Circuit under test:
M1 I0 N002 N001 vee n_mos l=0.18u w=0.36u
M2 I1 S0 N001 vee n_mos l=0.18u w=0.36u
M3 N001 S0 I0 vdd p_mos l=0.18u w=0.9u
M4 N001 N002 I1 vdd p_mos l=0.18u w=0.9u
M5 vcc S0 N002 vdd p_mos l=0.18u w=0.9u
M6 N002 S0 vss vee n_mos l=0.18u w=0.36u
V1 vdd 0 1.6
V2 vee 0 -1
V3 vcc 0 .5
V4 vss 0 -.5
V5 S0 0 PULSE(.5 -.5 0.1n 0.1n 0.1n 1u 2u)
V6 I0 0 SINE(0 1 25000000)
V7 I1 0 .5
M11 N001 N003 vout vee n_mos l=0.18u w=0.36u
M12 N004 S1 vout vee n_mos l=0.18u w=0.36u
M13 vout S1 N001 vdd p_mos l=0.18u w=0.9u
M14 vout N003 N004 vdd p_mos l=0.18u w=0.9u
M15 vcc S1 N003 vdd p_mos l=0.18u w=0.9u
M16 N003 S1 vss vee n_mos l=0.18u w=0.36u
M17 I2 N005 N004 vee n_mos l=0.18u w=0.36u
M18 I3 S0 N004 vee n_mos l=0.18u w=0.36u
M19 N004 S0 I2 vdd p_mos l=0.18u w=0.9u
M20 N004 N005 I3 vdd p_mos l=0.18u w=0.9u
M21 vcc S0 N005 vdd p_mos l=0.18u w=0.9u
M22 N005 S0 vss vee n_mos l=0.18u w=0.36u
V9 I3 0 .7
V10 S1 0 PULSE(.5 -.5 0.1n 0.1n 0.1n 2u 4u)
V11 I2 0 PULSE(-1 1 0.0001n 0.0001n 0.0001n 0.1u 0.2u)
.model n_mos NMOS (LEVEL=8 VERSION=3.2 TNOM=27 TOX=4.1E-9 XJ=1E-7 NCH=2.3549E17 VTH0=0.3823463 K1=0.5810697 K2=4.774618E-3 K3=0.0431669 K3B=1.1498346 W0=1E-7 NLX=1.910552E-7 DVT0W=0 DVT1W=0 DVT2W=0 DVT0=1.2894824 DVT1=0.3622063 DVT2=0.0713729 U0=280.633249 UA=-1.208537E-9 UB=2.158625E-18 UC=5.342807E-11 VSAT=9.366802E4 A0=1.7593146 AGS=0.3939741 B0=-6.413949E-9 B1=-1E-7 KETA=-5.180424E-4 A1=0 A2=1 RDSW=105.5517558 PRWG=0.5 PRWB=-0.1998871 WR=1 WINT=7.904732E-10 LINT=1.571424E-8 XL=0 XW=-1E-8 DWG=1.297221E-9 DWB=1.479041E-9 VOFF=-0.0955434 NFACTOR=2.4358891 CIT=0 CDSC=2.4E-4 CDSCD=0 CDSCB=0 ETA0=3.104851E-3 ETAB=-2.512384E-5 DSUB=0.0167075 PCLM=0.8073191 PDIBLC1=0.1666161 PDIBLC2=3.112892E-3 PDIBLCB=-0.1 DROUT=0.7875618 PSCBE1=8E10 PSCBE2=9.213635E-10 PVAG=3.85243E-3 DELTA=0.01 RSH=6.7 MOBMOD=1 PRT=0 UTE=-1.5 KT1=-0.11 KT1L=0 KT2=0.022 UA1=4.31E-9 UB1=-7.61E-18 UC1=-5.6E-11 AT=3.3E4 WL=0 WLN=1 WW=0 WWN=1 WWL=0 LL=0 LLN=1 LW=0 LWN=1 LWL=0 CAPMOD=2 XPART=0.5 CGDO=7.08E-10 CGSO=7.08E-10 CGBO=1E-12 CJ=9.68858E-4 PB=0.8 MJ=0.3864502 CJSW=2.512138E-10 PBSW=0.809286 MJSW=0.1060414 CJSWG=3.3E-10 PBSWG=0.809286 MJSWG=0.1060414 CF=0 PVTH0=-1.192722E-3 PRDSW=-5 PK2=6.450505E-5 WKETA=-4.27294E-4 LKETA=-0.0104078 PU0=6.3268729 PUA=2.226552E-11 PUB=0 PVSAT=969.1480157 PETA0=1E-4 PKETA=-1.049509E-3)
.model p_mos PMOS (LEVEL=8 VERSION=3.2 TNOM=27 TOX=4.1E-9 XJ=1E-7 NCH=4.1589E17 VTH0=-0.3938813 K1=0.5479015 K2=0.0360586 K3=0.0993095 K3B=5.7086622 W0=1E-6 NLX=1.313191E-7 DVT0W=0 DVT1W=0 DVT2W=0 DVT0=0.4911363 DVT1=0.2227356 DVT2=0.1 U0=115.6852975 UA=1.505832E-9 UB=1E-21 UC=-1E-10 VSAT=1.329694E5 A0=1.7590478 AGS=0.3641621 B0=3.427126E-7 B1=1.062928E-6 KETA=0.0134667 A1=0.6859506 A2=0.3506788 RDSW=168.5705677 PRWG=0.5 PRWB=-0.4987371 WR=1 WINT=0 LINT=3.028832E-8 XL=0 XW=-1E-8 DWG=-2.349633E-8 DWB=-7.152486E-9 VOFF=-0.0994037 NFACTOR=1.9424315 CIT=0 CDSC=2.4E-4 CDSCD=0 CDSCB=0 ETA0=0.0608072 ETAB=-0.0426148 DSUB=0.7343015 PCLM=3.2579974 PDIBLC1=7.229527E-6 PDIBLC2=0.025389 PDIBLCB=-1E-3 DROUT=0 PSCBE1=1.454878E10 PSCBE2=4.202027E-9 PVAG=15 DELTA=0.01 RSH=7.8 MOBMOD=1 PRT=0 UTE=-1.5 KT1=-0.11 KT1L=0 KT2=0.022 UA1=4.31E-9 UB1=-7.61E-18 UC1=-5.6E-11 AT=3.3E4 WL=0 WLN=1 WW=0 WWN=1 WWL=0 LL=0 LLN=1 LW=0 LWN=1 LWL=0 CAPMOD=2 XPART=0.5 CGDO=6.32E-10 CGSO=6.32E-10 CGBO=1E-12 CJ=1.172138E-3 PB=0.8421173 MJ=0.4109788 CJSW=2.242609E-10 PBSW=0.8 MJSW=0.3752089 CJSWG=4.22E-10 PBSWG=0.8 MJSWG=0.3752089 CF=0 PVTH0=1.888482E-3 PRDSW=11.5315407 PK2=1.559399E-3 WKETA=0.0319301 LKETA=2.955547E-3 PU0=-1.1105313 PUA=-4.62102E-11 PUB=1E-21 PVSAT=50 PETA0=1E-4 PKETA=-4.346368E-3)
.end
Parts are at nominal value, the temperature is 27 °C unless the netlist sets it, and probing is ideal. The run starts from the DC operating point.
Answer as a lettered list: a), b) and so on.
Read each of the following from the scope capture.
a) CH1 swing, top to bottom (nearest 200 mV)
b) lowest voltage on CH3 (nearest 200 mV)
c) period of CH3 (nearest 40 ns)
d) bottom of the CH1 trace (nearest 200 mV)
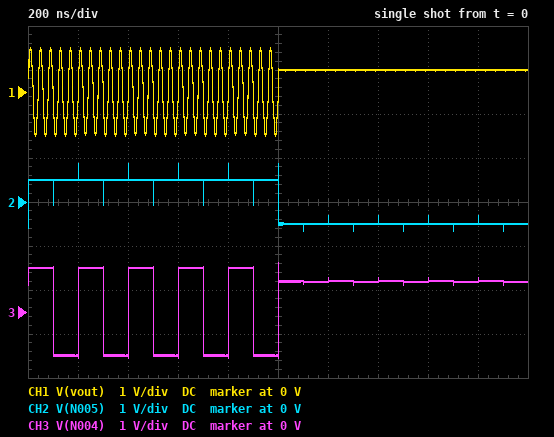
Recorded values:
a) 2.0 V
b) -1.0 V
c) 200 ns
d) -1.0 V
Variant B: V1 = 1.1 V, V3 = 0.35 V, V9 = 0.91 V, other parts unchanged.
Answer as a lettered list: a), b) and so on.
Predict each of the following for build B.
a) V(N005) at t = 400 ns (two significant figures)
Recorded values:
a) 350 mV
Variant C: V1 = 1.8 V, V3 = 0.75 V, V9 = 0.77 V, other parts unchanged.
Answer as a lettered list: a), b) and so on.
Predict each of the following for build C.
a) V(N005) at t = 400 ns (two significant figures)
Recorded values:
a) 750 mV
